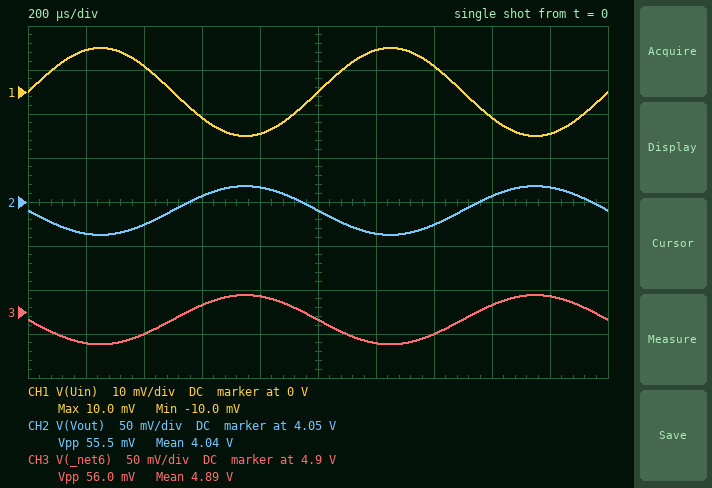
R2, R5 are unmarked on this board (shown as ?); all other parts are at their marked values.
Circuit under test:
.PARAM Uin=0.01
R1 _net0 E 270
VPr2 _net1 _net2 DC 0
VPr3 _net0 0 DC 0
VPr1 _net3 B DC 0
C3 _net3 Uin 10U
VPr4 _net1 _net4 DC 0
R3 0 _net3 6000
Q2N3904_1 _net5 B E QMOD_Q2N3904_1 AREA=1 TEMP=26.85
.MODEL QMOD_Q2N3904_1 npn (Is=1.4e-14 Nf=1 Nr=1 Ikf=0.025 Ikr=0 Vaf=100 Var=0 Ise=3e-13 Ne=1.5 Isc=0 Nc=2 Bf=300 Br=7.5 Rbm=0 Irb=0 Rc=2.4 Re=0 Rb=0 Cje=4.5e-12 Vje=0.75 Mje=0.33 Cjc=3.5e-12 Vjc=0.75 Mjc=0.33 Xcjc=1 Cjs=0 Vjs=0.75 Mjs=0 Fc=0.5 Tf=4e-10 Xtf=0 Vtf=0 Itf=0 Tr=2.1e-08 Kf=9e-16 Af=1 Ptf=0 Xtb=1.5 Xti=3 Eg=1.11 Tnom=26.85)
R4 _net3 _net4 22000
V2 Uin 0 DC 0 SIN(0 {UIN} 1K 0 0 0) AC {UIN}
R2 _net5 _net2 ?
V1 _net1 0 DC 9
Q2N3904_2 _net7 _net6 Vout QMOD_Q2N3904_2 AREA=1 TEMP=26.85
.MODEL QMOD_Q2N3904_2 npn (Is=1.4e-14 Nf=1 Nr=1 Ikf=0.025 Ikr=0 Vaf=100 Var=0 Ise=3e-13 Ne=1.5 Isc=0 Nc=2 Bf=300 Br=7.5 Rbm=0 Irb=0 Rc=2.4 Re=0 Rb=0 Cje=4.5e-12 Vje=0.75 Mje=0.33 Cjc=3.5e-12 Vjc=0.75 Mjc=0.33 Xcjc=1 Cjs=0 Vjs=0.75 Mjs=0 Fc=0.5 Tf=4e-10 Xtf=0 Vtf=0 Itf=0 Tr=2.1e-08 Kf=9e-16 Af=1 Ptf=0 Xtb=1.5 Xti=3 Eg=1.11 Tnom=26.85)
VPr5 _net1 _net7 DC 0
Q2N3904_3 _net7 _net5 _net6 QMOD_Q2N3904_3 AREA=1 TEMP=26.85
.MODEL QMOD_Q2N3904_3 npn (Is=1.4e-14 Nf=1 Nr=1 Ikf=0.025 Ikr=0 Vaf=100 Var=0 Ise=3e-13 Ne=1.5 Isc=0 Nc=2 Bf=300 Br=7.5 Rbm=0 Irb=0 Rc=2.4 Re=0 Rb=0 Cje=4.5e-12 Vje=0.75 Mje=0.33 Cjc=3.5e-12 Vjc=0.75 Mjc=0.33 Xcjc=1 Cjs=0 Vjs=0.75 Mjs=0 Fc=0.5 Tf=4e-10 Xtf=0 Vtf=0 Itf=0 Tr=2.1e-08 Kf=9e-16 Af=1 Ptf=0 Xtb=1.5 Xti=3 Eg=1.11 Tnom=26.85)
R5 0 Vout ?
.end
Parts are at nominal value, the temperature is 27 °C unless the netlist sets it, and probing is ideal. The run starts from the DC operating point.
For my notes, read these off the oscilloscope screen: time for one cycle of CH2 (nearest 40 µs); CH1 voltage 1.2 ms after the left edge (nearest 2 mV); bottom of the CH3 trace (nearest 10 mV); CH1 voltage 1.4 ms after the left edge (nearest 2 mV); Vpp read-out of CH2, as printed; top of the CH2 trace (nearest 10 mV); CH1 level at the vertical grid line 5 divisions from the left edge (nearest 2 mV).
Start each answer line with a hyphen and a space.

- 1.00 ms
- 10 mV
- 4.86 V
- 6 mV
- 55.5 mV
- 4.07 V
- 0 V
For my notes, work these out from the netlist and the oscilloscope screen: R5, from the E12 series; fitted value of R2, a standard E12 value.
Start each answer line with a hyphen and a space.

- 15 Ω
- 820 Ω
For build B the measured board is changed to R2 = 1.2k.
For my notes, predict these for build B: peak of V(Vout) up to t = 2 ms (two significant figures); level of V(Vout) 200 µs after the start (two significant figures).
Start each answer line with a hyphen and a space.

- 2.6 V
- 2.5 V
